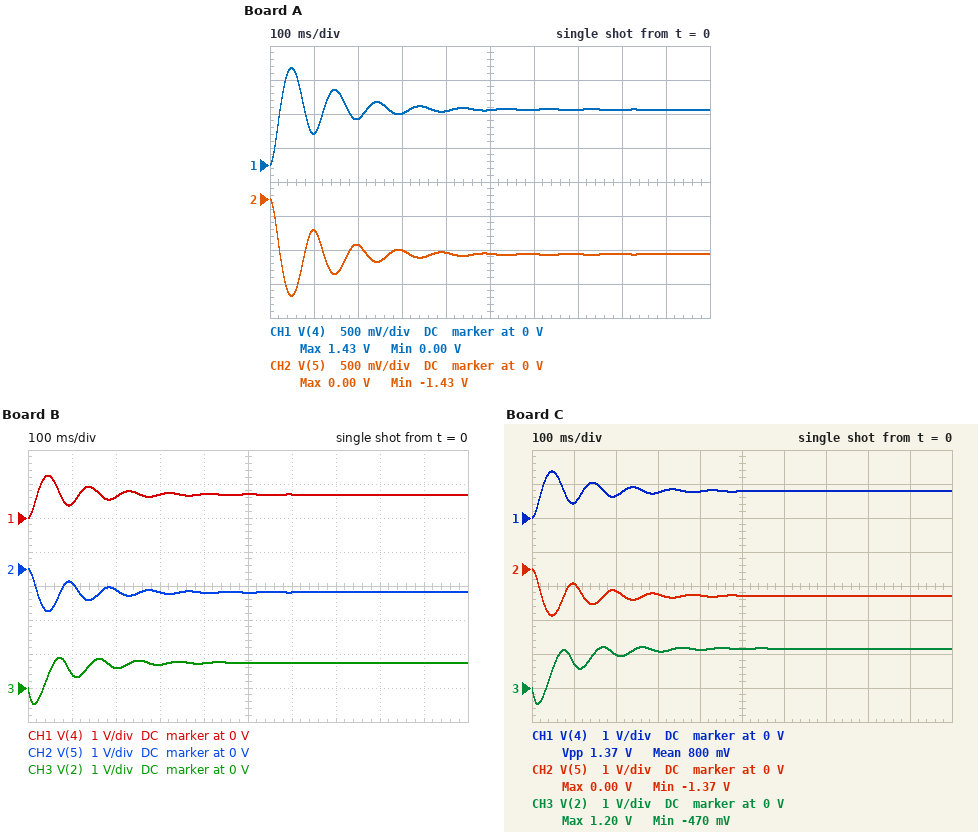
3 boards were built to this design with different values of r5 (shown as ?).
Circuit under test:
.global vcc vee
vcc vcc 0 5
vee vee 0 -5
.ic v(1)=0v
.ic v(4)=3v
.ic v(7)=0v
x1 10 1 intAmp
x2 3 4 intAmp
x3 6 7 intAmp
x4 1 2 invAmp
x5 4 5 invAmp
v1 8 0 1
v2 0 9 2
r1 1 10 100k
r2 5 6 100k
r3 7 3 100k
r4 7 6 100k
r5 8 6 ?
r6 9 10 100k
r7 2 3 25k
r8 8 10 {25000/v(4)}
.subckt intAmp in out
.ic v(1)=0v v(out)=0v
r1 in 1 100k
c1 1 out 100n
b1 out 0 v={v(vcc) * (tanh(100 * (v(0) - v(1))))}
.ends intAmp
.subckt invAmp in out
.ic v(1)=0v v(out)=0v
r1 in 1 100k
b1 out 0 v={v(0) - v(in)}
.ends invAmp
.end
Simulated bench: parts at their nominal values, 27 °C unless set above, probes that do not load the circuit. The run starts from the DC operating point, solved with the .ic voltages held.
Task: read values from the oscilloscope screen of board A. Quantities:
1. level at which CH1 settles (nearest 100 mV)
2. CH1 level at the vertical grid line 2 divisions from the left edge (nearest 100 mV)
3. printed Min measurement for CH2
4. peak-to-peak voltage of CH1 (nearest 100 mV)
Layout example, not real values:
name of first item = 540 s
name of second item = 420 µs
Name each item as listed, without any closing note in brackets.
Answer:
level at which CH1 settles = 800 mV
CH1 level at the vertical grid line 2 divisions from the left edge = 700 mV
printed Min measurement for CH2 = -1.43 V
peak-to-peak voltage of CH1 = 1.4 V
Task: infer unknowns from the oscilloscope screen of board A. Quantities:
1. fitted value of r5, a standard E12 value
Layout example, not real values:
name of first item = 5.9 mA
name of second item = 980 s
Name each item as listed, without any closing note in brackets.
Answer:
fitted value of r5, a standard E12 value = 15 kΩ
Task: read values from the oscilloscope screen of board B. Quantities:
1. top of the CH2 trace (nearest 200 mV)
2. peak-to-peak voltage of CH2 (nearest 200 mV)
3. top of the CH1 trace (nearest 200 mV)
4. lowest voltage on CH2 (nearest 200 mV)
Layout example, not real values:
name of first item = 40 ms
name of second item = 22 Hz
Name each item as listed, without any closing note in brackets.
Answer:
top of the CH2 trace = 0 V
peak-to-peak voltage of CH2 = 1.2 V
top of the CH1 trace = 1.2 V
lowest voltage on CH2 = -1.2 V
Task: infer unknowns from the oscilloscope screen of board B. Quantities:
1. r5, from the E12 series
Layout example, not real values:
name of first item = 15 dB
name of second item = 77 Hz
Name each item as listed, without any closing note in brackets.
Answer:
r5, from the E12 series = 27 kΩ
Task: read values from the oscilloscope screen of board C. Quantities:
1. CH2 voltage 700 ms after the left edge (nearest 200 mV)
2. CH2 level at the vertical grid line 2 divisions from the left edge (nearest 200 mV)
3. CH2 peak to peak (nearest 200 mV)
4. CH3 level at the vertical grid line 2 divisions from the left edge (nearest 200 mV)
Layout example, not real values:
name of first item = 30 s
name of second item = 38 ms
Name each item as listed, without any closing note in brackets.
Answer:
CH2 voltage 700 ms after the left edge = -800 mV
CH2 level at the vertical grid line 2 divisions from the left edge = -600 mV
CH2 peak to peak = 1.4 V
CH3 level at the vertical grid line 2 divisions from the left edge = 1.0 V
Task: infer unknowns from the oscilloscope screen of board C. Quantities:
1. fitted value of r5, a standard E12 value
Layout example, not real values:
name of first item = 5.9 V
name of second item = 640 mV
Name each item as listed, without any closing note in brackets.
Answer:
fitted value of r5, a standard E12 value = 18 kΩ
